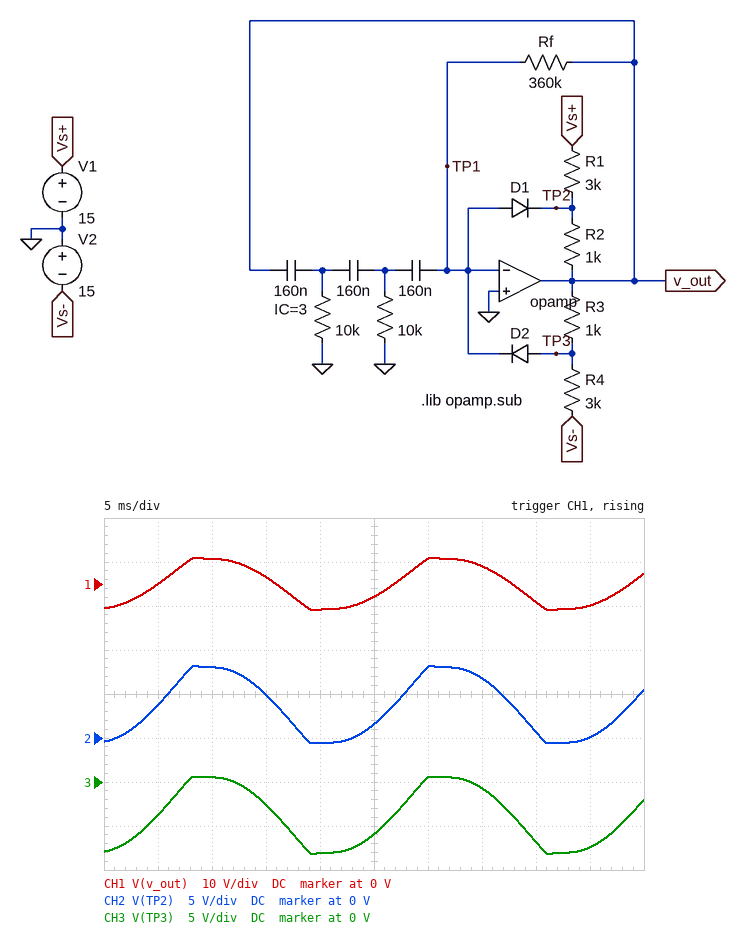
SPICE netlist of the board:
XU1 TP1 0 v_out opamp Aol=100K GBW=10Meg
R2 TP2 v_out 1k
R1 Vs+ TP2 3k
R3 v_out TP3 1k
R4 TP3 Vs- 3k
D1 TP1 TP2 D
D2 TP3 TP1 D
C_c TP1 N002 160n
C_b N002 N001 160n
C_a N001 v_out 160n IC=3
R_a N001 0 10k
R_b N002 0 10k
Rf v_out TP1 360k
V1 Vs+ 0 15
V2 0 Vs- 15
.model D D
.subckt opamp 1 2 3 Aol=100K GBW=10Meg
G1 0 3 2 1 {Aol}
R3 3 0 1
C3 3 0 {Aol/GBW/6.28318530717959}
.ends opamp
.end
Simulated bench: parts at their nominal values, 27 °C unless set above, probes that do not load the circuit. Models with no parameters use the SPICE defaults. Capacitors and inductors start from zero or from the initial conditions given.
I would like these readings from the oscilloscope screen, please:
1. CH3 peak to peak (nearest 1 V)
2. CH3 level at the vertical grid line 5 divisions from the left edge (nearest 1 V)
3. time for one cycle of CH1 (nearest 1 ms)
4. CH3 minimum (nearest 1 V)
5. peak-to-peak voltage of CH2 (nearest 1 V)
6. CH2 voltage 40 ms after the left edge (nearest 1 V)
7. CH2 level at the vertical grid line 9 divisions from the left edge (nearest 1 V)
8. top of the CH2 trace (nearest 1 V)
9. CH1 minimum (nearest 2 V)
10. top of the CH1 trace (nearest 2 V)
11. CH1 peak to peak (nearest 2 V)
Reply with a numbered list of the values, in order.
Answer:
1. 9 V
2. -6 V
3. 22 ms
4. -8 V
5. 9 V
6. 1 V
7. 0 V
8. 8 V
9. -6 V
10. 6 V
11. 12 V
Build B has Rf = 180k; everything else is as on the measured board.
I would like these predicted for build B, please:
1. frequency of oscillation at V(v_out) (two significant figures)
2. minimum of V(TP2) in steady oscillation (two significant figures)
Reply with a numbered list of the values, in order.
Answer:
1. 53 Hz
2. -580 mV
